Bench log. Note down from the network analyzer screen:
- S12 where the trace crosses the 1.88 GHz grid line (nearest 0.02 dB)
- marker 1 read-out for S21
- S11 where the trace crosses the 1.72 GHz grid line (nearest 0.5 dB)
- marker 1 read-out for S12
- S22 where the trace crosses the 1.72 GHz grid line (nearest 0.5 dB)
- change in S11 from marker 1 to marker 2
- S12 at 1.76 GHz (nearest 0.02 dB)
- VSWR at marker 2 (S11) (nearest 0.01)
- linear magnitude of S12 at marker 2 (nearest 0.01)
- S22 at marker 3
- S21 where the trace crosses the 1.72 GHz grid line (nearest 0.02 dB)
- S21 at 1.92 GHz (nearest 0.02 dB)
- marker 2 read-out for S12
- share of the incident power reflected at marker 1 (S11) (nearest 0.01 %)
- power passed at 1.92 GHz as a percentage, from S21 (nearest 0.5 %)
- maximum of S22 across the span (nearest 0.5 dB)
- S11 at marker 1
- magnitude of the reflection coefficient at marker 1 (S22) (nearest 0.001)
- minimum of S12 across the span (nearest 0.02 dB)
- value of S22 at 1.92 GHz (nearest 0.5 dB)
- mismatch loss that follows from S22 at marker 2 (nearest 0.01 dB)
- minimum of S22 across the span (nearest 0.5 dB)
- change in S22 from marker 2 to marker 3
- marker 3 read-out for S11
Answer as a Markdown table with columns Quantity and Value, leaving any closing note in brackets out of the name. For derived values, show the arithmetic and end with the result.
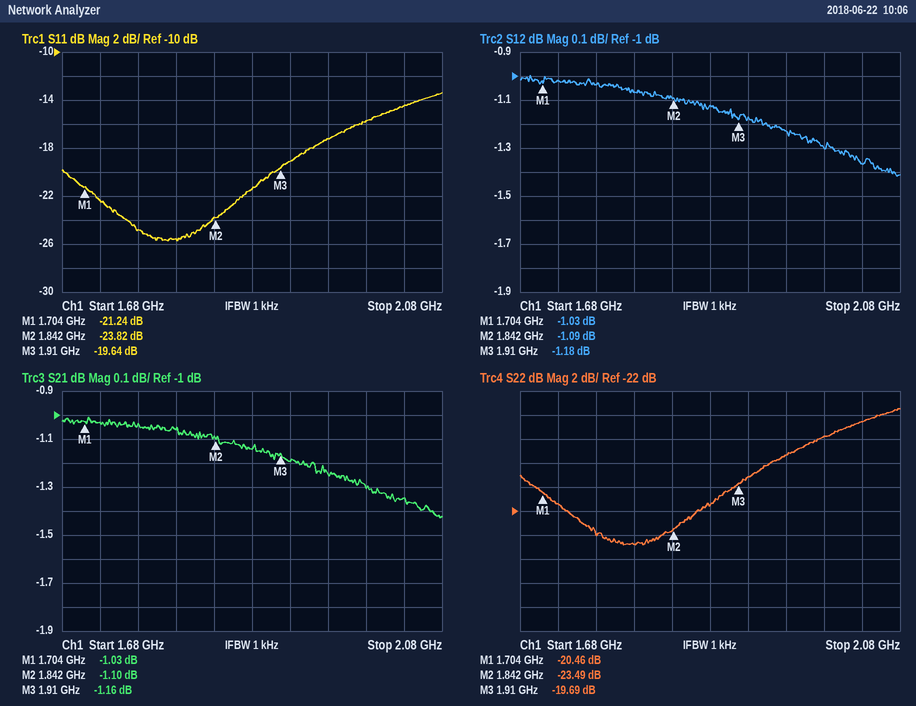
| Quantity | Value |
|---|---|
| S12 where the trace crosses the 1.88 GHz grid line | -1.12 dB |
| marker 1 read-out for S21 | -1.03 dB |
| S11 where the trace crosses the 1.72 GHz grid line | -22.5 dB |
| marker 1 read-out for S12 | -1.03 dB |
| S22 where the trace crosses the 1.72 GHz grid line | -21.5 dB |
| change in S11 from marker 1 to marker 2 | -23.82 − (-21.24) = -2.58 dB |
| S12 at 1.76 GHz | -1.04 dB |
| VSWR at marker 2 (S11) | (1 + 0.0644)/(1 − 0.0644) ≈ 1.14 |
| linear magnitude of S12 at marker 2 | 10^(-1.09/20) ≈ 0.88 |
| S22 at marker 3 | -19.69 dB |
| S21 where the trace crosses the 1.72 GHz grid line | -1.04 dB |
| S21 at 1.92 GHz | -1.20 dB |
| marker 2 read-out for S12 | -1.09 dB |
| share of the incident power reflected at marker 1 (S11) | 10^(-21.24/10) ≈ 0.75 % |
| power passed at 1.92 GHz as a percentage, from S21 | 10^(-1.2/10) ≈ 75.9 %, so 76.0 % to the nearest 0.5 % |
| maximum of S22 across the span | -13.5 dB |
| S11 at marker 1 | -21.24 dB |
| magnitude of the reflection coefficient at marker 1 (S22) | 10^(-20.46/20) ≈ 0.095 |
| minimum of S12 across the span | -1.42 dB |
| value of S22 at 1.92 GHz | -19.0 dB |
| mismatch loss that follows from S22 at marker 2 | −10 log10(1 − 10^(-23.49/10)) ≈ 0.02 dB |
| minimum of S22 across the span | -25.0 dB |
| change in S22 from marker 2 to marker 3 | -19.69 − (-23.49) = 3.80 dB |
| marker 3 read-out for S11 | -19.64 dB |
